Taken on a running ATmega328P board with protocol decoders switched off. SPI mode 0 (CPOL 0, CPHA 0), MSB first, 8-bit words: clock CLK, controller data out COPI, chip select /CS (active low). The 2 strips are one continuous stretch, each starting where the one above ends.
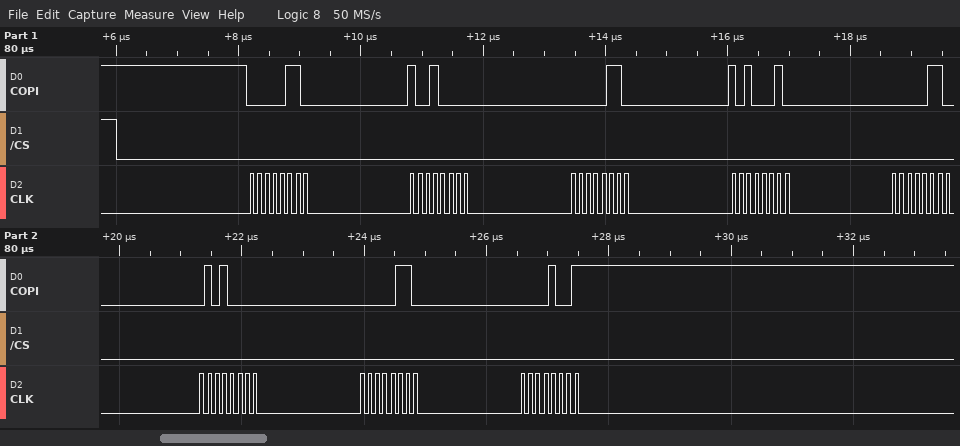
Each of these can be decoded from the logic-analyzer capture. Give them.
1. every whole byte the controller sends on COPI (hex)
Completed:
06 90 06 A2 06 50 06 09
